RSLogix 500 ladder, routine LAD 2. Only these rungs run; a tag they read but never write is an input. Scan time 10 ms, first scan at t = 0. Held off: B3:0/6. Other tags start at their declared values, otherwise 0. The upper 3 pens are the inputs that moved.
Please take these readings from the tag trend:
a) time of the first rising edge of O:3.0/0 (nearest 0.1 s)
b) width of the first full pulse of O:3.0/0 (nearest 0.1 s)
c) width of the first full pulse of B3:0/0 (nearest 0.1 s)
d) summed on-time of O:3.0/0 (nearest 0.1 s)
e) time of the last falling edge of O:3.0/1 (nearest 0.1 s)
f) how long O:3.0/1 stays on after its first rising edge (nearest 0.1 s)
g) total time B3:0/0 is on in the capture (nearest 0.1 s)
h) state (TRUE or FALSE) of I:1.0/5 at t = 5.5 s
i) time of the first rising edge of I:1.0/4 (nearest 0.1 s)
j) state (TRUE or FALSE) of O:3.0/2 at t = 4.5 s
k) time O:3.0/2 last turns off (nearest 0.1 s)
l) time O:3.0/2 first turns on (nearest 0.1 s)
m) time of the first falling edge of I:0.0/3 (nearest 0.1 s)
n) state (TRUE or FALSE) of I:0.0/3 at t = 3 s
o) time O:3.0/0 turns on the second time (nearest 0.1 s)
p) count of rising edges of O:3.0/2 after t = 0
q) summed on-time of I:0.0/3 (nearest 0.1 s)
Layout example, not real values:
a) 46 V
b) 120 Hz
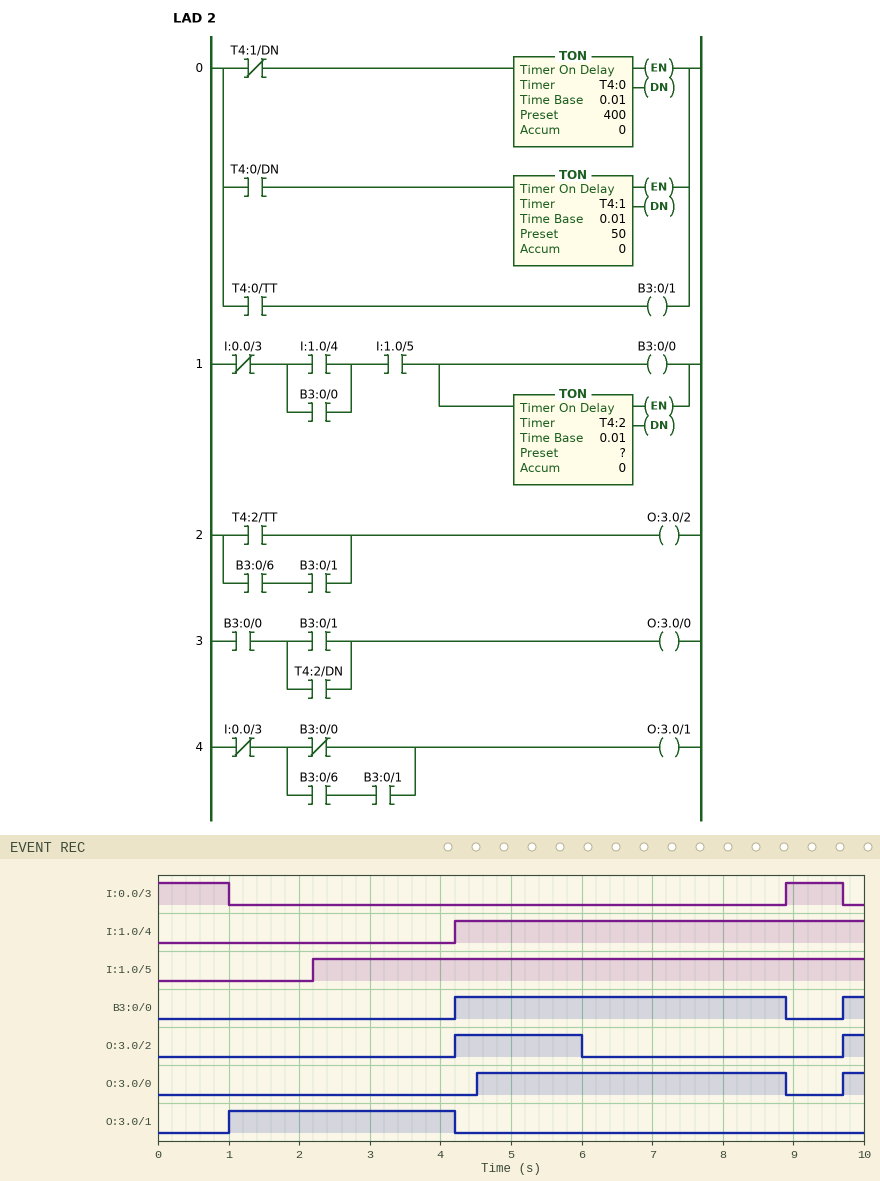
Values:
a) 4.5 s
b) 4.4 s
c) 4.7 s
d) 4.7 s
e) 4.2 s
f) 3.2 s
g) 5.0 s
h) TRUE
i) 4.2 s
j) TRUE
k) 6.0 s
l) 4.2 s
m) 1.0 s
n) FALSE
o) 9.7 s
p) 2
q) 1.8 s
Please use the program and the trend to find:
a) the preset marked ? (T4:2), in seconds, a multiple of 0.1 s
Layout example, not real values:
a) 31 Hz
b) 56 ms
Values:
a) 1.8 s
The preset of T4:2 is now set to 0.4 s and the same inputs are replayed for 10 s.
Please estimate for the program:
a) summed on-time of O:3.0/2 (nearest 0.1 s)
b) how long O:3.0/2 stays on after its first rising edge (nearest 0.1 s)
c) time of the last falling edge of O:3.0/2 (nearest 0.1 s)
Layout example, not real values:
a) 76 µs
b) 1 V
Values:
a) 0.7 s
b) 0.4 s
c) 4.6 s
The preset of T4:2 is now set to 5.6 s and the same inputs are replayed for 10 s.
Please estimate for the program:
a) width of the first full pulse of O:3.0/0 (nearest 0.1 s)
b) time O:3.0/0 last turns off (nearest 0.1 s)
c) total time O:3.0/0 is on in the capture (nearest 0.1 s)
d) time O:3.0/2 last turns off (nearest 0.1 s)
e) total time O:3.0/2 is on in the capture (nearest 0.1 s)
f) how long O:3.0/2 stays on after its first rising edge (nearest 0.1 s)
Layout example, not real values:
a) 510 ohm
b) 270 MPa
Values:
a) 4.0 s
b) 8.5 s
c) 4.3 s
d) 8.9 s
e) 5.0 s
f) 4.7 s
